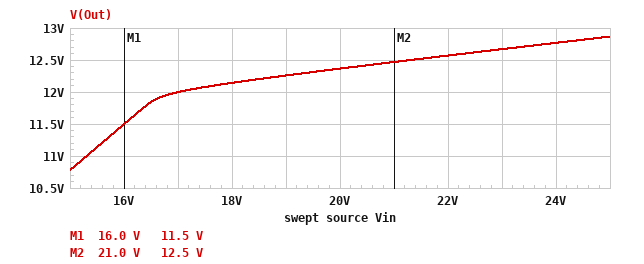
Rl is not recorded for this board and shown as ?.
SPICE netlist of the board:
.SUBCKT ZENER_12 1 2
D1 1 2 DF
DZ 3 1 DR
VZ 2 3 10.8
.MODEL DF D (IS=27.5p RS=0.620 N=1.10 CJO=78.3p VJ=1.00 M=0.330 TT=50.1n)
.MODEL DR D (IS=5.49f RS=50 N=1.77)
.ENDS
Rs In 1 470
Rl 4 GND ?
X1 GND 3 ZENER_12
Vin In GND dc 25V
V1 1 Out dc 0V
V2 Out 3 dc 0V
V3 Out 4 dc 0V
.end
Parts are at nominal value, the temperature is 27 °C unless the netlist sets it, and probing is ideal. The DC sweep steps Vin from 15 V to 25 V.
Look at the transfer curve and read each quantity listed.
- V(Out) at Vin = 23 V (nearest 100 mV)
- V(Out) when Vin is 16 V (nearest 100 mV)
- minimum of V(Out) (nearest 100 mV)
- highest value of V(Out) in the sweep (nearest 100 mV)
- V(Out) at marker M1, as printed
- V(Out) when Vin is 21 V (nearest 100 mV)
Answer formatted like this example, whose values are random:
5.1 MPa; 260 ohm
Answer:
12.7 V; 11.5 V; 10.8 V; 12.9 V; 11.5 V; 12.5 V
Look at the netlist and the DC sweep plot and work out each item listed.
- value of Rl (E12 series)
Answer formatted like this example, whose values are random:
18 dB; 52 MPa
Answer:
1.2 kΩ
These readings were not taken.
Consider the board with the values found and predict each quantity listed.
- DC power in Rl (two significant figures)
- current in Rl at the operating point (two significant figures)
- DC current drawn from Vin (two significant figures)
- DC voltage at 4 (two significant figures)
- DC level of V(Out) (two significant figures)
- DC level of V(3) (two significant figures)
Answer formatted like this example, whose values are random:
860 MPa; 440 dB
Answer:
140 mW; 11 mA; 26 mA; 13 V; 13 V; 13 V
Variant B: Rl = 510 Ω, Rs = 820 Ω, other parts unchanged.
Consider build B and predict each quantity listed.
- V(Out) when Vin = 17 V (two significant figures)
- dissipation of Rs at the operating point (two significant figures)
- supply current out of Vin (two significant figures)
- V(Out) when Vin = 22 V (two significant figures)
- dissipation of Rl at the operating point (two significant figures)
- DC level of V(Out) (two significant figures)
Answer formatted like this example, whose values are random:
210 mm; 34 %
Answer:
6.5 V; 290 mW; 19 mA; 8.4 V; 180 mW; 9.6 V
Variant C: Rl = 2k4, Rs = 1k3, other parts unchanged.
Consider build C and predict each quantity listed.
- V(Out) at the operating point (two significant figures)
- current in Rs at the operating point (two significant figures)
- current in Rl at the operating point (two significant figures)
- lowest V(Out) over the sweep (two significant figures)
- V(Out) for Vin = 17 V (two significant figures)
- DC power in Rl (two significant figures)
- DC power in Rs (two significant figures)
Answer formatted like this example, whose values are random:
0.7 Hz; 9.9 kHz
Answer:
12 V; 9.8 mA; 5.1 mA; 9.7 V; 11 V; 63 mW; 120 mW
